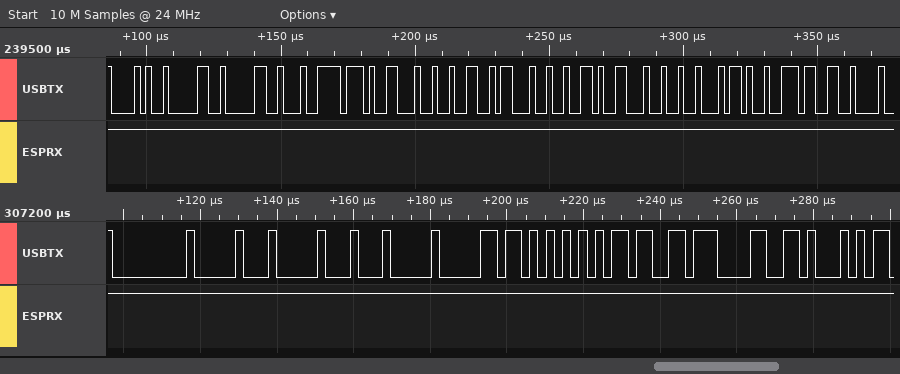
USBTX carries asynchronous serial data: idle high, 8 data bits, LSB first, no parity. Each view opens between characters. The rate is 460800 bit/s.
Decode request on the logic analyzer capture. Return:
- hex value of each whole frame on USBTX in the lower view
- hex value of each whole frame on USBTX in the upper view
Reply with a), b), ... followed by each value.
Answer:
a) 00, 10, 10, 04, B0, 55, 9B, 87, 16
b) 28, 30, 30, E4, 97, 24, A6, 24, 96, 24, A2, C9, 33
